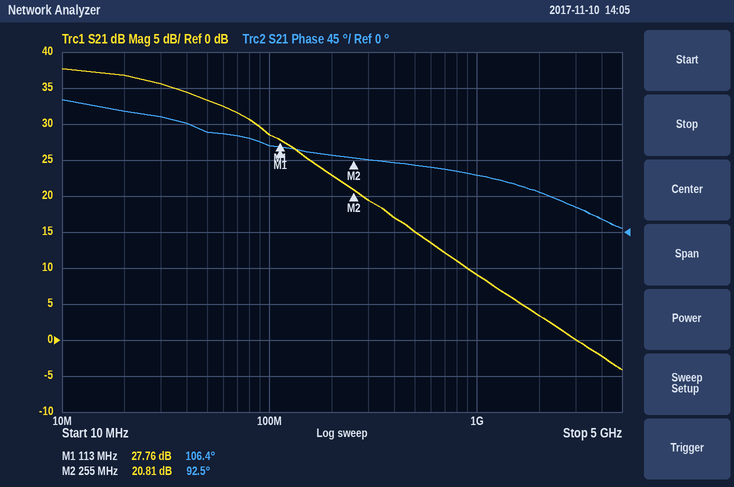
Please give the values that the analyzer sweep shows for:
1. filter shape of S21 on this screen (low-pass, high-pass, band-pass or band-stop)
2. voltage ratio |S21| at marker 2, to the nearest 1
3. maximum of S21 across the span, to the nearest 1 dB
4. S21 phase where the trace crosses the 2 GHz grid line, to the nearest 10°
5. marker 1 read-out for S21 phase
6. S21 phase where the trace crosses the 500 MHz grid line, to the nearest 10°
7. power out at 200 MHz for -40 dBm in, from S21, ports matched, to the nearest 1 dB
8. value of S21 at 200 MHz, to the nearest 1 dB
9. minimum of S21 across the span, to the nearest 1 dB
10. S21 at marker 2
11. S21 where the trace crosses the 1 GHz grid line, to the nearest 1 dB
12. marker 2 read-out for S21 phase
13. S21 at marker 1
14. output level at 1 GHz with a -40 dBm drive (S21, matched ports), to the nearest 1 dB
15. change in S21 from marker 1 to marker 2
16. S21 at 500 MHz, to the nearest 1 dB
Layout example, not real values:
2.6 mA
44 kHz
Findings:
low-pass
11
38 dB
50°
106.4°
80°
-17 dBm
23 dB
-4 dB
20.81 dB
9 dB
92.5°
27.76 dB
-31 dBm
-6.95 dB
15 dB
